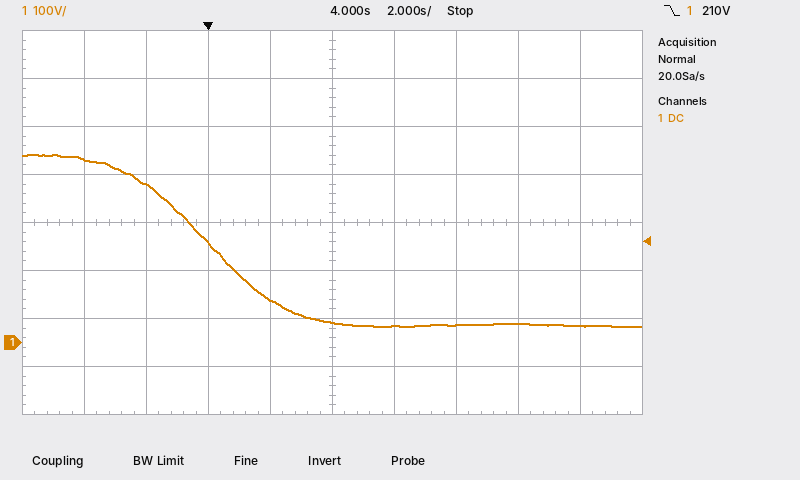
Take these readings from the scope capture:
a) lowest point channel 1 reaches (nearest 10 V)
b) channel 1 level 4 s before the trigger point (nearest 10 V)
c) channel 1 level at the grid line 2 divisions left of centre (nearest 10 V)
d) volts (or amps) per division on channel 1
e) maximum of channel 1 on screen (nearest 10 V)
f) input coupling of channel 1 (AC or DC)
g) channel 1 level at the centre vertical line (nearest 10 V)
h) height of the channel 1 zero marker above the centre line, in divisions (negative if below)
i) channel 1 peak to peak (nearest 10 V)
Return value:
30 V
380 V
210 V
100 V
390 V
DC
40 V
-2.5 div
360 V
